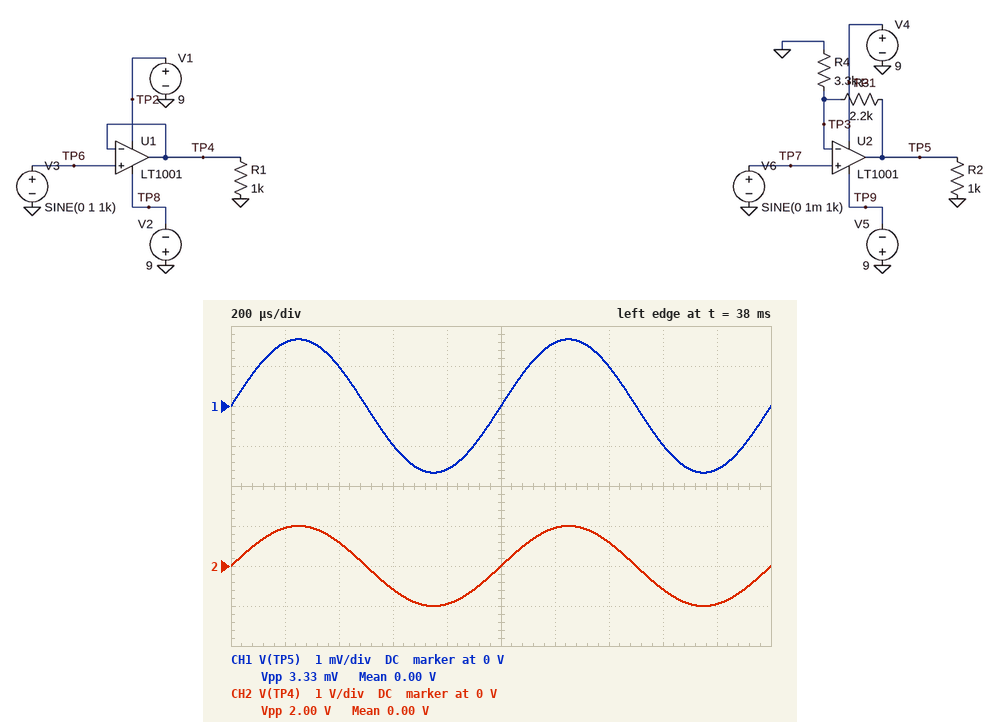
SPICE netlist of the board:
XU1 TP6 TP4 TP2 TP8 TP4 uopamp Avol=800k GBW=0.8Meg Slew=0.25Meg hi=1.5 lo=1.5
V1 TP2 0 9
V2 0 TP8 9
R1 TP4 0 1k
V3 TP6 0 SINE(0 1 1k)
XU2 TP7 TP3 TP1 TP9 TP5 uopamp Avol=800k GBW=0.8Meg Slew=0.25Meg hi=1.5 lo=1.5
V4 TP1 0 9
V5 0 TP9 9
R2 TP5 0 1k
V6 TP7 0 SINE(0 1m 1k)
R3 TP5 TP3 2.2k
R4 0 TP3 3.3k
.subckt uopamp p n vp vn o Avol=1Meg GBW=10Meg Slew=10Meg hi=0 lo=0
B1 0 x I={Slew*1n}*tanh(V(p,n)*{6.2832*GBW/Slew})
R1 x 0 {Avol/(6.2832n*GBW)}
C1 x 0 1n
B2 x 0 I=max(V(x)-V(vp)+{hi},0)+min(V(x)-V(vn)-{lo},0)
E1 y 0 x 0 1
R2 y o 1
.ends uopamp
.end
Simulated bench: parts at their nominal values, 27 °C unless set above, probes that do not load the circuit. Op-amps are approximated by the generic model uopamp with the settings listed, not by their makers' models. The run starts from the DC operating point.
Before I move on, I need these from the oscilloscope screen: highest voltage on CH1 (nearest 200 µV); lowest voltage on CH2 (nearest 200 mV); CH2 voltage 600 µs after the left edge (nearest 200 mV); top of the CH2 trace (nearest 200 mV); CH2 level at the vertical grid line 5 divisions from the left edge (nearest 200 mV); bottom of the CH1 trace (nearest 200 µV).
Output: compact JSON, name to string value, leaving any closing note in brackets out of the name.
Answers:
{"highest voltage on CH1": "1.6 mV", "lowest voltage on CH2": "-1.0 V", "CH2 voltage 600 µs after the left edge": "-600 mV", "top of the CH2 trace": "1.0 V", "CH2 level at the vertical grid line 5 divisions from the left edge": "0 V", "bottom of the CH1 trace": "-1.6 mV"}
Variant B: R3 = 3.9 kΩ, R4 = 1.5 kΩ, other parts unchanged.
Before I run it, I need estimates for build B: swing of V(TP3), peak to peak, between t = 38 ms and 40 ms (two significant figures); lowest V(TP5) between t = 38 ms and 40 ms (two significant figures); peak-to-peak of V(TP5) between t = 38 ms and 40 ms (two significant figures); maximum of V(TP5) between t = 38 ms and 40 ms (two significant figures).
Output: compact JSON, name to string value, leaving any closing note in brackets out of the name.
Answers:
{"swing of V(TP3), peak to peak, between t = 38 ms and 40 ms": "2.0 mV", "lowest V(TP5) between t = 38 ms and 40 ms": "-3.6 mV", "peak-to-peak of V(TP5) between t = 38 ms and 40 ms": "7.2 mV", "maximum of V(TP5) between t = 38 ms and 40 ms": "3.6 mV"}
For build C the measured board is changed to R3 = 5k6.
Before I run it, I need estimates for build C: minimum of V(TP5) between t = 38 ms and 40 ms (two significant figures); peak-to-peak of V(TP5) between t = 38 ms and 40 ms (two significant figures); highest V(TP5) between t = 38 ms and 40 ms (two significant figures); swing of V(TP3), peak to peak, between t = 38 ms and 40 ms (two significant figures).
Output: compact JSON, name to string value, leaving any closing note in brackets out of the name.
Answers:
{"minimum of V(TP5) between t = 38 ms and 40 ms": "-2.7 mV", "peak-to-peak of V(TP5) between t = 38 ms and 40 ms": "5.4 mV", "highest V(TP5) between t = 38 ms and 40 ms": "2.7 mV", "swing of V(TP3), peak to peak, between t = 38 ms and 40 ms": "2.0 mV"}
